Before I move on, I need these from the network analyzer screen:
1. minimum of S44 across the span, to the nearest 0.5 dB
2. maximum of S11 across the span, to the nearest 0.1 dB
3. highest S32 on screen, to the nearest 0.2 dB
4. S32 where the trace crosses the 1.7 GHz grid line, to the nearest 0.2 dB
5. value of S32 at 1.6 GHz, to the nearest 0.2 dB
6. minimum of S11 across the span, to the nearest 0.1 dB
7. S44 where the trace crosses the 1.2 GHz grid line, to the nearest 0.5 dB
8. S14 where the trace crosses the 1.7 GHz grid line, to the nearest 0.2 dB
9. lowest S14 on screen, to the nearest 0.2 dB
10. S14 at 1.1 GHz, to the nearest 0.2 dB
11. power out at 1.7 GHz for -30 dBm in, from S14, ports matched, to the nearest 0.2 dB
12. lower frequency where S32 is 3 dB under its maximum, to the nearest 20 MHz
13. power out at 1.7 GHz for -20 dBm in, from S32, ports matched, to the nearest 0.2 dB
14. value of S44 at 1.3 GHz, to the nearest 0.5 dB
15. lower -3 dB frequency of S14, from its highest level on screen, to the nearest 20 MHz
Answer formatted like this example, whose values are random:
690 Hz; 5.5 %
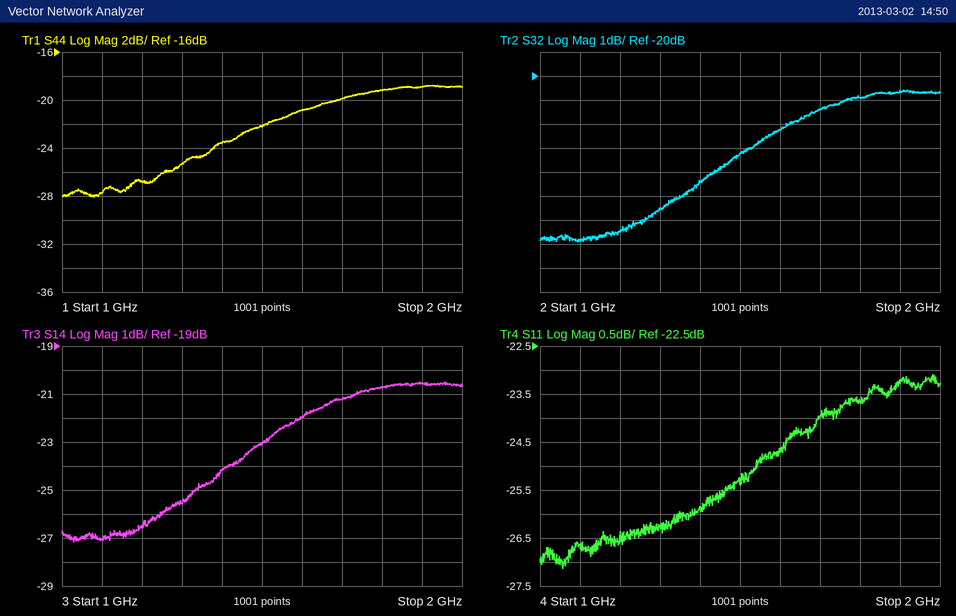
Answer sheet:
-28.0 dB; -23.1 dB; -20.6 dB; -21.4 dB; -22.2 dB; -27.1 dB; -27.0 dB; -21.2 dB; -27.2 dB; -27.0 dB; -51.2 dBm; 1.48 GHz; -41.4 dBm; -25.5 dB; 1.46 GHz
